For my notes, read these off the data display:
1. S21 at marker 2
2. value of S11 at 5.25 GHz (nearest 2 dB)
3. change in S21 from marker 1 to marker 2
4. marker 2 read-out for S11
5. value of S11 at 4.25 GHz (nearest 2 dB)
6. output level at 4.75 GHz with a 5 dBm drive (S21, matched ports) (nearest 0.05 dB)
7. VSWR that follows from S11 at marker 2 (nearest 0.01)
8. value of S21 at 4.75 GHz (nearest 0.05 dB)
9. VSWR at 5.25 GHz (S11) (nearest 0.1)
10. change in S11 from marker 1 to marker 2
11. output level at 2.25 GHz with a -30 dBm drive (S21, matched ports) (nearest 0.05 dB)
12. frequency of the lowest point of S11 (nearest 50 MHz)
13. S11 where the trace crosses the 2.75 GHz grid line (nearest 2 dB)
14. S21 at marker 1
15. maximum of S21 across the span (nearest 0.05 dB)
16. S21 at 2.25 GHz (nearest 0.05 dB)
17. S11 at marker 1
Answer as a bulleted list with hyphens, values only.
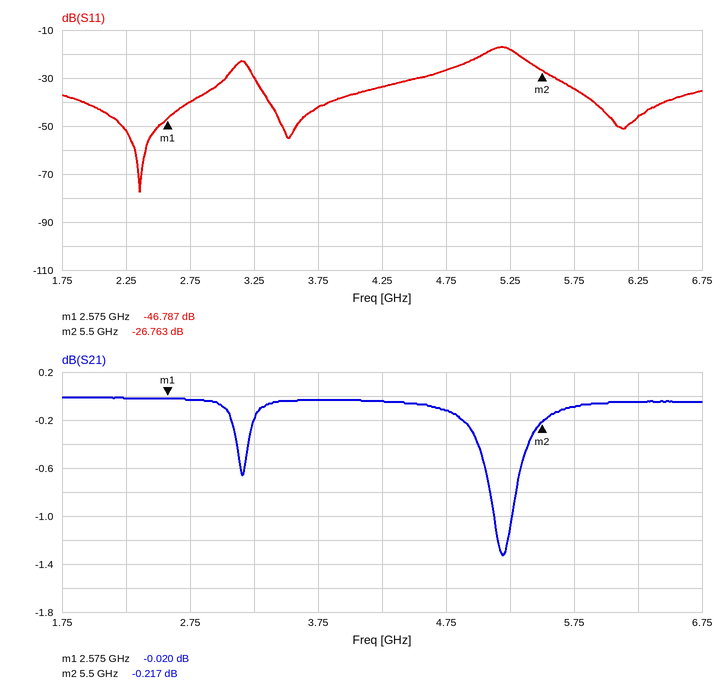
- -0.217 dB
- -18 dB
- -0.197 dB
- -26.763 dB
- -34 dB
- 4.90 dBm
- 1.10
- -0.10 dB
- 1.3
- 20.024 dB
- -30.00 dBm
- 2.35 GHz
- -40 dB
- -0.020 dB
- 0.00 dB
- 0.00 dB
- -46.787 dB
